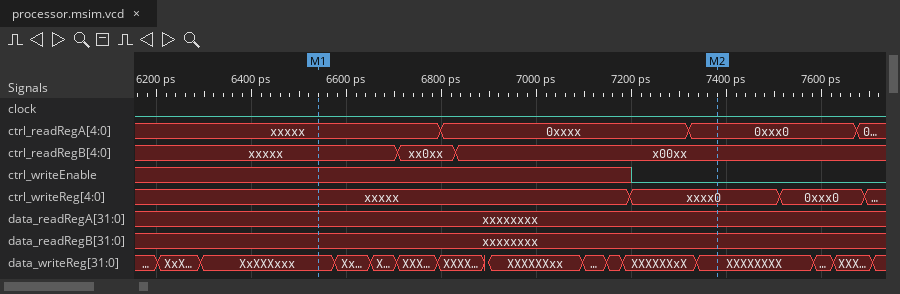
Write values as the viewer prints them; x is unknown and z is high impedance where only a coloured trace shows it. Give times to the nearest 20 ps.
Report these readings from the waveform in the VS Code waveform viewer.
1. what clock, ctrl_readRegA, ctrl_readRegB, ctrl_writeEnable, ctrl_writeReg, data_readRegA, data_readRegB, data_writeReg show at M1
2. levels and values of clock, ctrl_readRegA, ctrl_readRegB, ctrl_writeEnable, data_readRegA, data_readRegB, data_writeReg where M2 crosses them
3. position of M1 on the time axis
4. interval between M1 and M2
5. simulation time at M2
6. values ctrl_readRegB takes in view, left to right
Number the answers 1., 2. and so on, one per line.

1. clock=0, ctrl_readRegA=xxxxx, ctrl_readRegB=xxxxx, ctrl_writeEnable=x, ctrl_writeReg=xxxxx, data_readRegA=xxxxxxxx, data_readRegB=xxxxxxxx, data_writeReg=XxXXXxxx
2. clock=0, ctrl_readRegA=0xxx0, ctrl_readRegB=x00xx, ctrl_writeEnable=0, data_readRegA=xxxxxxxx, data_readRegB=xxxxxxxx, data_writeReg=XXXXXXXX
3. 6540 ps
4. 840 ps
5. 7380 ps
6. xxxxx, xx0xx, x00xx
